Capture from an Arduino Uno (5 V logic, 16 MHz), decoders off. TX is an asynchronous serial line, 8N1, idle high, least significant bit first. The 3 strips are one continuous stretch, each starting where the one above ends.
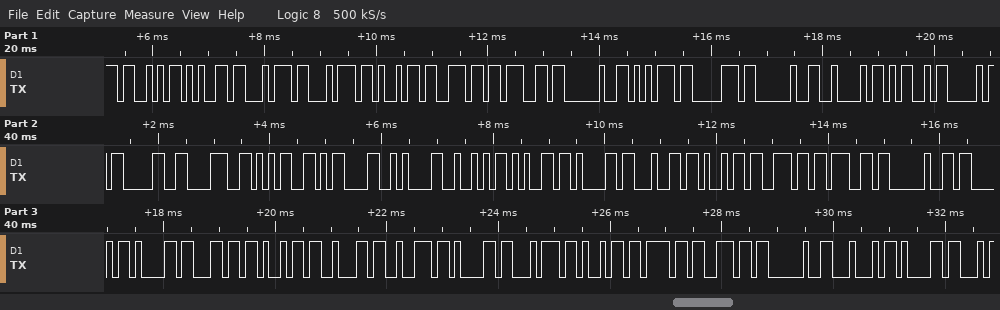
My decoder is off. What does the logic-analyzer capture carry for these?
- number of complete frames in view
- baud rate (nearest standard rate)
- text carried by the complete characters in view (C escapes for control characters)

41
9600 baud
"Setting up BMP085\r\nReading Calibration Da"
